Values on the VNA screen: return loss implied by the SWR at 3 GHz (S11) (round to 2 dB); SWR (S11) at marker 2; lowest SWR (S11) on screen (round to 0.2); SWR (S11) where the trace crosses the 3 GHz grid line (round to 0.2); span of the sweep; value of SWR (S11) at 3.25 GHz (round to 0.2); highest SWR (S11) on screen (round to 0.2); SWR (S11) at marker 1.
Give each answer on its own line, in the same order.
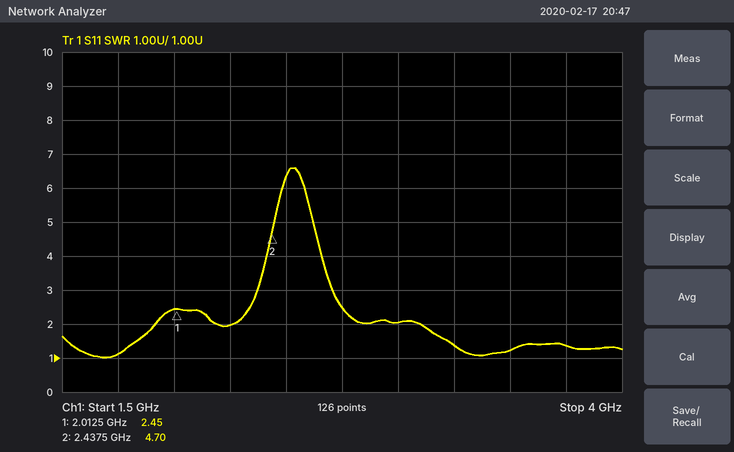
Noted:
10 dB
4.70
1.0
2.0
2.5 GHz
1.4
6.6
2.45
